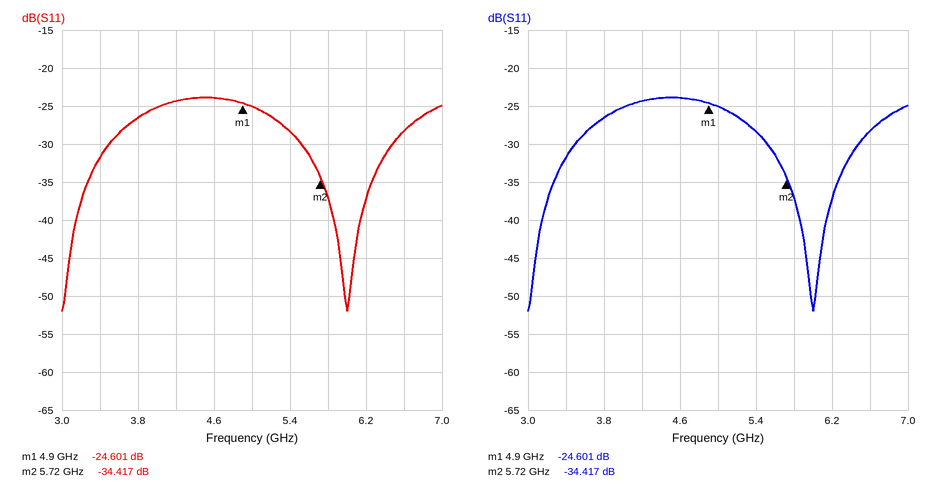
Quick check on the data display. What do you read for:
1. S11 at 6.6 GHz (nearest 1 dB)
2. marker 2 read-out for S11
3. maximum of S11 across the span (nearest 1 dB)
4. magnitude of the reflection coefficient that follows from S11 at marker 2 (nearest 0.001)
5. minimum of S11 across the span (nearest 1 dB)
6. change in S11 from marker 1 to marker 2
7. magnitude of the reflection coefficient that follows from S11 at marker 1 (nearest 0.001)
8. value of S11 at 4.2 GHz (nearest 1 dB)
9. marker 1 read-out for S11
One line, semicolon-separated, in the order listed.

-28 dB; -34.417 dB; -24 dB; 0.019; -52 dB; -9.816 dB; 0.059; -24 dB; -24.601 dB
